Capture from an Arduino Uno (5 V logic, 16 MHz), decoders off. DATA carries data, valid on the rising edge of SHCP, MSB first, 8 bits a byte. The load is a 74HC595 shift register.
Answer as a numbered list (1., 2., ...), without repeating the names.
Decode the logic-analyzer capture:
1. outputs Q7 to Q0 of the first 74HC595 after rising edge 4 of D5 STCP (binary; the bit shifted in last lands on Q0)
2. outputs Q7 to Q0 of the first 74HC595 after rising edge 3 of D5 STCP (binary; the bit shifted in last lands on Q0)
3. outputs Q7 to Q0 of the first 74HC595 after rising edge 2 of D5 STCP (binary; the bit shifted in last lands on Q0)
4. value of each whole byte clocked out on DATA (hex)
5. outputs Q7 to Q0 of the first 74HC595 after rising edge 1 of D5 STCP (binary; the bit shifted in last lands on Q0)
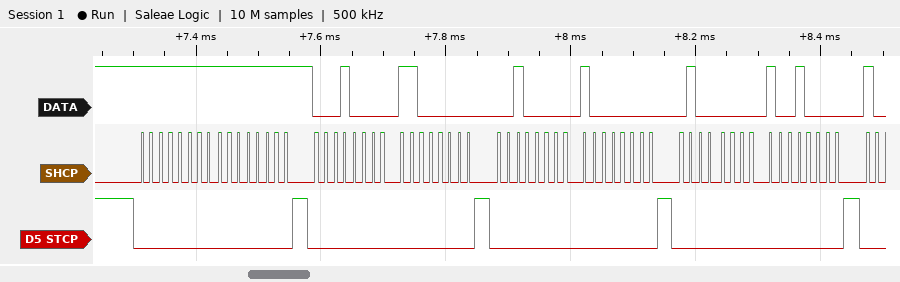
1. 10010000
2. 10000000
3. 11000000
4. FF FF 10 C0 20 80 40 90
5. 11111111
